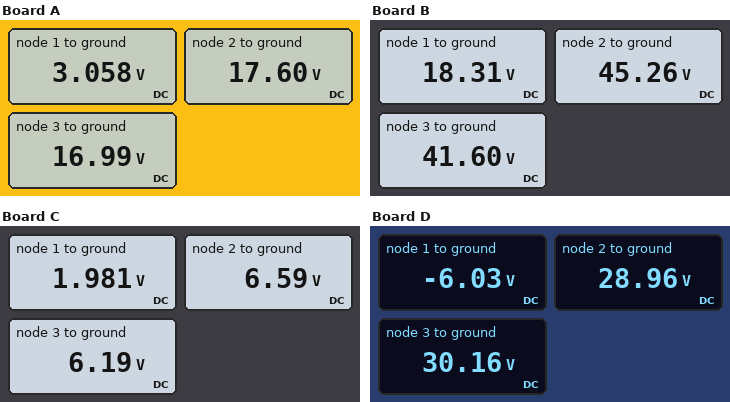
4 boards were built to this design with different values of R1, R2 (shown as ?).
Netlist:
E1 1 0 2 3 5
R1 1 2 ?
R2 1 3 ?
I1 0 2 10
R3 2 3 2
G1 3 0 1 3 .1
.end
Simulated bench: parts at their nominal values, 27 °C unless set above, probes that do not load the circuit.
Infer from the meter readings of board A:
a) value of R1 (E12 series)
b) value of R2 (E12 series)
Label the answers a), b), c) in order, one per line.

a) 1.5 Ω
b) 8.2 Ω
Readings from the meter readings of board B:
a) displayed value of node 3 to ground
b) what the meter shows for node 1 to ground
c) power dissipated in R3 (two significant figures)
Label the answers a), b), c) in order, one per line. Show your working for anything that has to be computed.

a) 41.60 V
b) 18.31 V
c) (45.26 V - 41.6 V)^2 / 2 Ω = 6.7 W
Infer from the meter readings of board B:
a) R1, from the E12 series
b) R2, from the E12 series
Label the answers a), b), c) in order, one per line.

a) 3.3 Ω
b) 5.6 Ω
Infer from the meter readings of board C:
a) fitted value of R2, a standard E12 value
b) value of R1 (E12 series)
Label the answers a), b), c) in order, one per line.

a) 6.8 Ω
b) 0.47 Ω
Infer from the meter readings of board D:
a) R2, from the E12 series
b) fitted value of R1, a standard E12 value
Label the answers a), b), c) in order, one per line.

a) 12 Ω
b) 3.3 Ω
